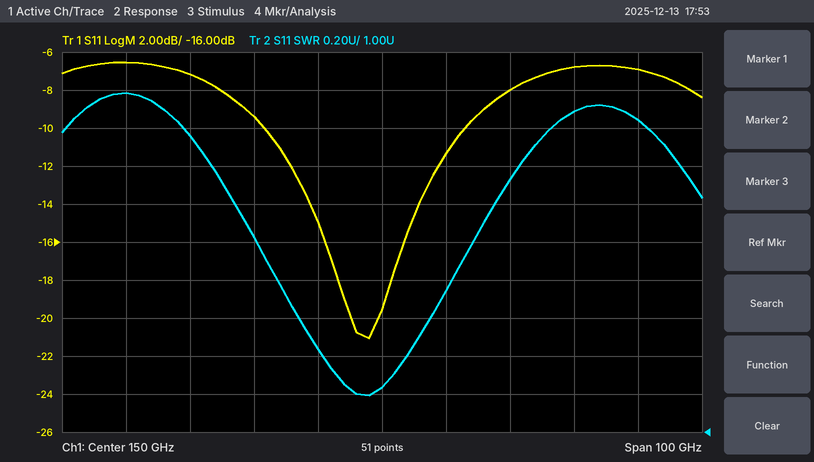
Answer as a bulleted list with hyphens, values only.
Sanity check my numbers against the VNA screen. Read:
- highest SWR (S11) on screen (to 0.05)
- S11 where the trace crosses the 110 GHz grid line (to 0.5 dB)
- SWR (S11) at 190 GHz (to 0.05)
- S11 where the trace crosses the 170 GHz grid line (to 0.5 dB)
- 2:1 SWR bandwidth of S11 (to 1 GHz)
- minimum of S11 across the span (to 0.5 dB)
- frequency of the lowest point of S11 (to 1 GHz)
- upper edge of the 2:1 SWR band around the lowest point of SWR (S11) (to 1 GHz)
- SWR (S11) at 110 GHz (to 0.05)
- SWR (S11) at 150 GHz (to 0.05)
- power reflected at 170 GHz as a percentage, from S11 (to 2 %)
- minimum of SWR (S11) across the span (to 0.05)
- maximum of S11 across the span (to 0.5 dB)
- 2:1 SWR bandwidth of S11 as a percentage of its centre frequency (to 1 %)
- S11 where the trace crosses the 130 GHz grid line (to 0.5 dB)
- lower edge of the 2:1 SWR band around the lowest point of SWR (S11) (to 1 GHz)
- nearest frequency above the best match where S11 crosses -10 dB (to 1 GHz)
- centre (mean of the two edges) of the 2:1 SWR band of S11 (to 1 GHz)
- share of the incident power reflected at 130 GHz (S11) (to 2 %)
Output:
- 2.80
- -6.5 dB
- 2.65
- -8.0 dB
- 34 GHz
- -21.0 dB
- 148 GHz
- 164 GHz
- 2.80
- 1.25
- 16 %
- 1.20
- -6.5 dB
- 23 %
- -9.5 dB
- 130 GHz
- 163 GHz
- 147 GHz
- 12 %
